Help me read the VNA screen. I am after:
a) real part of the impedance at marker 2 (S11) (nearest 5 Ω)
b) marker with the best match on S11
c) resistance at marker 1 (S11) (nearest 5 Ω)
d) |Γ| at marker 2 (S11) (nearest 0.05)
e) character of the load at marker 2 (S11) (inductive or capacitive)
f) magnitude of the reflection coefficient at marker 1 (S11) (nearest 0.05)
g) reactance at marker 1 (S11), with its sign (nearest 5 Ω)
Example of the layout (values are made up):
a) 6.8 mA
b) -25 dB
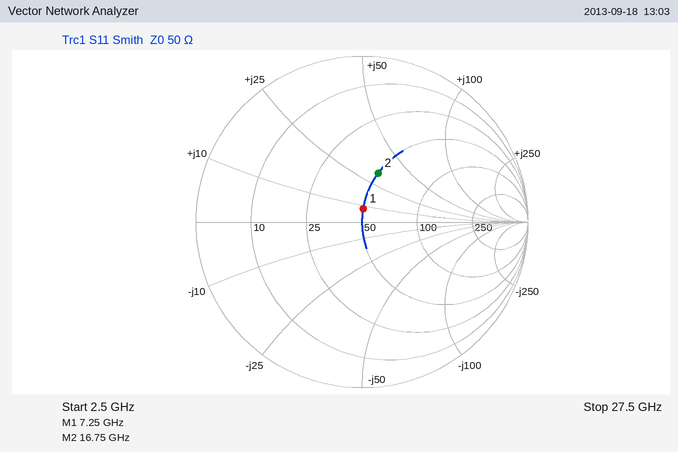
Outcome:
a) 50 Ω
b) marker 1
c) 50 Ω
d) 0.30
e) inductive
f) 0.10
g) +10 Ω
